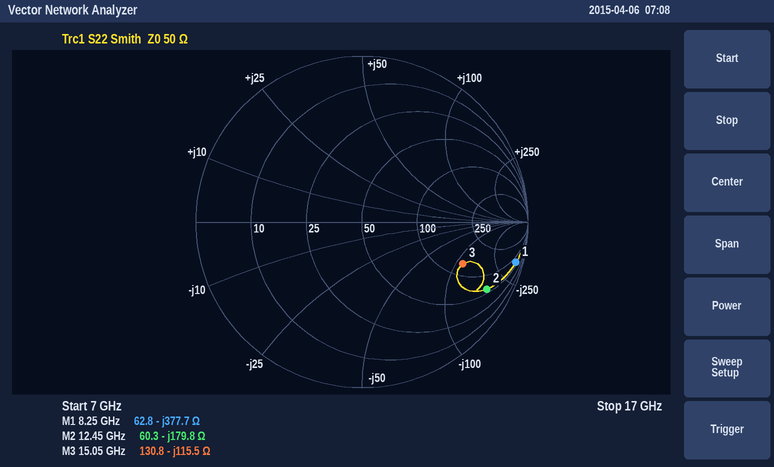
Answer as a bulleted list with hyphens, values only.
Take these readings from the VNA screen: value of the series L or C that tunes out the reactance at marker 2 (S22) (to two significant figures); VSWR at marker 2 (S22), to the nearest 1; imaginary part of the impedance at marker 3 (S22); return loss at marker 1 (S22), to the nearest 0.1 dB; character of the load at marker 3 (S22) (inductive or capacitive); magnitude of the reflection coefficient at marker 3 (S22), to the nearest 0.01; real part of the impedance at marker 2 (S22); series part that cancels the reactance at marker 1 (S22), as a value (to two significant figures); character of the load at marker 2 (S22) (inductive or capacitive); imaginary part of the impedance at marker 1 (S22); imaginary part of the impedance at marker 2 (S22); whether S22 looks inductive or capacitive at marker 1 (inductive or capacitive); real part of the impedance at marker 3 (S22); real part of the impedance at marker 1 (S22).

- 2.3 nH
- 13
- -115.5 Ω
- 0.4 dB
- capacitive
- 0.66
- 60.3 Ω
- 7.3 nH
- capacitive
- -377.7 Ω
- -179.8 Ω
- capacitive
- 130.8 Ω
- 62.8 Ω
